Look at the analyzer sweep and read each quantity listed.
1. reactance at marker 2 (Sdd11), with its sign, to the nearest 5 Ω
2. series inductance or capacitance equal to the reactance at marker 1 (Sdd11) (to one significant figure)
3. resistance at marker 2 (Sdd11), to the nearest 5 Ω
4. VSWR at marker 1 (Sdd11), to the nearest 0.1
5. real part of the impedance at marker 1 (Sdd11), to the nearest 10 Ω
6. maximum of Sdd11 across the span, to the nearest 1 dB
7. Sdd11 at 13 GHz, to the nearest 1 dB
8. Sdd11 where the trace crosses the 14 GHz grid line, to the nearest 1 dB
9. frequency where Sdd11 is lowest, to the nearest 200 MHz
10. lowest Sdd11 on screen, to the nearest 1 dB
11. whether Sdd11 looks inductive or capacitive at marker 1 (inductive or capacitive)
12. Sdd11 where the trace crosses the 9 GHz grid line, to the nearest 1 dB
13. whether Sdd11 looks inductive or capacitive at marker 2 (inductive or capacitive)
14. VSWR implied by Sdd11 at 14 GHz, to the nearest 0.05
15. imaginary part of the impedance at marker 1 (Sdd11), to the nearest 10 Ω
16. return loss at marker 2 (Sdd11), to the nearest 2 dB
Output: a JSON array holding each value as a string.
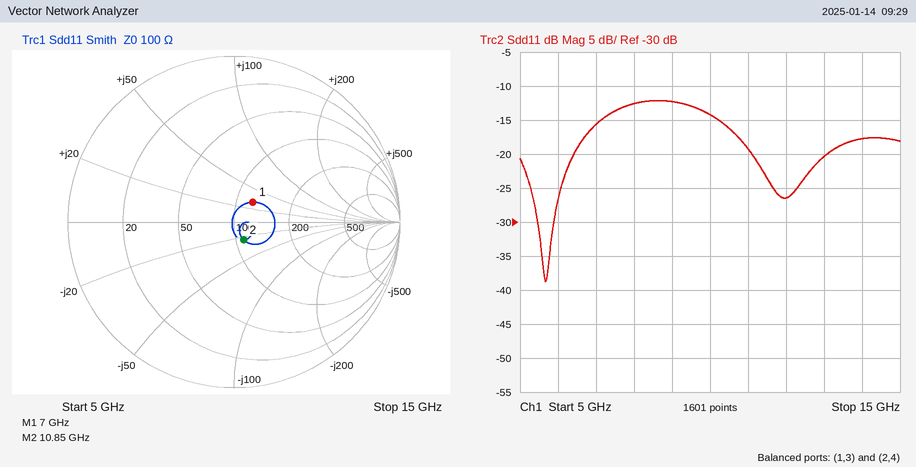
["-25 Ω", "700 pH", "110 Ω", "1.4", "120 Ω", "-12 dB", "-20 dB", "-18 dB", "5.6 GHz", "-39 dB", "inductive", "-12 dB", "capacitive", "1.30", "+30 Ω", "18 dB"]
